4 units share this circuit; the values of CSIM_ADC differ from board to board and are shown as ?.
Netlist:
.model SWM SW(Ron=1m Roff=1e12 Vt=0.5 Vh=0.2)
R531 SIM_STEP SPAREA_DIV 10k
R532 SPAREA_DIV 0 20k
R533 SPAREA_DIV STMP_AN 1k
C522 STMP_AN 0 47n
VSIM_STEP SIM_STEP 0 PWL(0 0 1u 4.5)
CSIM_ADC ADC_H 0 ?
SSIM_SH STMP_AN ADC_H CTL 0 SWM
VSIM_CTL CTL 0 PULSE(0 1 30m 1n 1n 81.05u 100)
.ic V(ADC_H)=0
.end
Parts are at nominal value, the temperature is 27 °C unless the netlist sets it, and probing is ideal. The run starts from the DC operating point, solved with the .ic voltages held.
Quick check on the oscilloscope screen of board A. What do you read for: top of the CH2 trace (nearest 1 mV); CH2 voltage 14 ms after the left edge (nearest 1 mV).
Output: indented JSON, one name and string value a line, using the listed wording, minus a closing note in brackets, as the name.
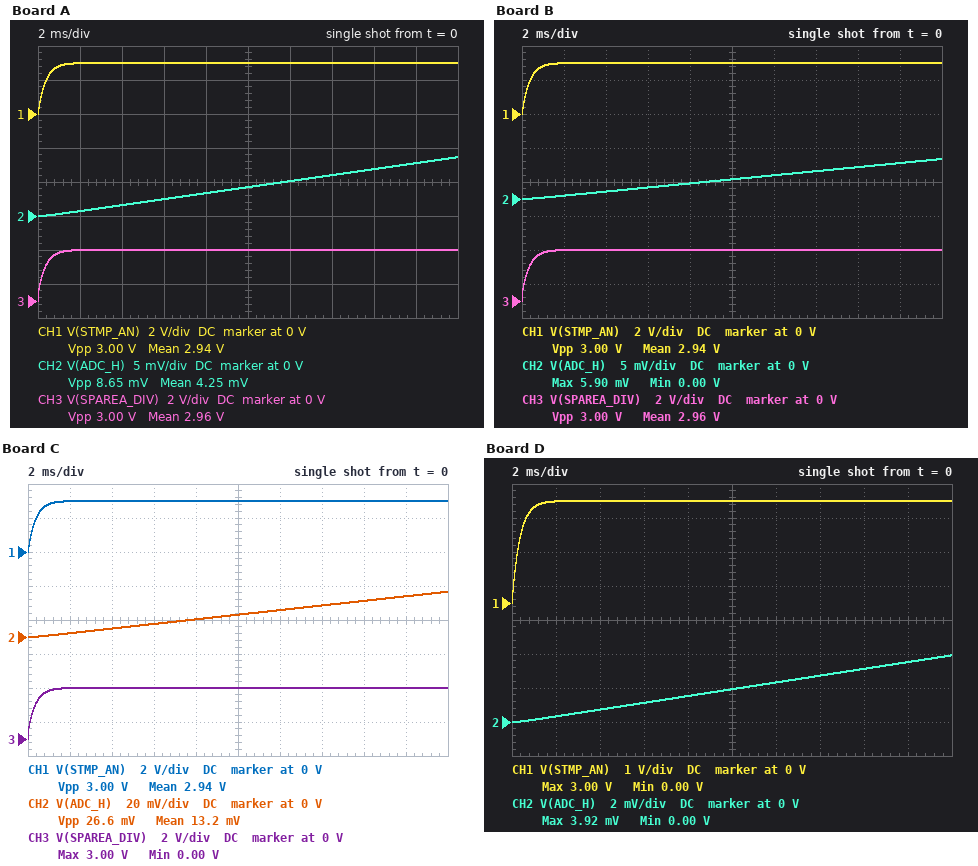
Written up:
{
  "top of the CH2 trace": "9 mV",
  "CH2 voltage 14 ms after the left edge": "6 mV"
}
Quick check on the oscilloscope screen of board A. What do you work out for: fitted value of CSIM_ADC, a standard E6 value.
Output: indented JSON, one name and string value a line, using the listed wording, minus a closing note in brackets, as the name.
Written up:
{
  "fitted value of CSIM_ADC, a standard E6 value": "6.8 pF"
}
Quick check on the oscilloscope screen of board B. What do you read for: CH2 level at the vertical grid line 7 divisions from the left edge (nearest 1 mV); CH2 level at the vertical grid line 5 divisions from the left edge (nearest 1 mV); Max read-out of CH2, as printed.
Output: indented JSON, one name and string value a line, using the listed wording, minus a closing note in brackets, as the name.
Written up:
{
  "CH2 level at the vertical grid line 7 divisions from the left edge": "4 mV",
  "CH2 level at the vertical grid line 5 divisions from the left edge": "3 mV",
  "Max read-out of CH2, as printed": "5.90 mV"
}
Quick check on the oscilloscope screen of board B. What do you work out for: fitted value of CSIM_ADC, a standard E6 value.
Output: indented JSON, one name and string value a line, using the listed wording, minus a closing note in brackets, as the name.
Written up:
{
  "fitted value of CSIM_ADC, a standard E6 value": "10 pF"
}
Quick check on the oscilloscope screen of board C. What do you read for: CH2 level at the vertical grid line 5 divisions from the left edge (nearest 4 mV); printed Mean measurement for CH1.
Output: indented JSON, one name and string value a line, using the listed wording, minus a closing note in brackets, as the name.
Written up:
{
  "CH2 level at the vertical grid line 5 divisions from the left edge": "12 mV",
  "printed Mean measurement for CH1": "2.94 V"
}
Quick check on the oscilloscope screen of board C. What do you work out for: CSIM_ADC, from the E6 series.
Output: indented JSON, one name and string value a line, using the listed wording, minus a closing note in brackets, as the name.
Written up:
{
  "CSIM_ADC, from the E6 series": "2.2 pF"
}
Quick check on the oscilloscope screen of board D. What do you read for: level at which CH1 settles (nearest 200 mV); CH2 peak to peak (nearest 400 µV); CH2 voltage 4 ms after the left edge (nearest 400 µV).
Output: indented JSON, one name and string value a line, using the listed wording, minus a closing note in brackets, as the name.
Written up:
{
  "level at which CH1 settles": "3.0 V",
  "CH2 peak to peak": "4.0 mV",
  "CH2 voltage 4 ms after the left edge": "800 µV"
}
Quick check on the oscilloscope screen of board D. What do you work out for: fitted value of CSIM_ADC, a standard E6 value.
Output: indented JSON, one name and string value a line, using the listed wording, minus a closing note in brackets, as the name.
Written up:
{
  "fitted value of CSIM_ADC, a standard E6 value": "15 pF"
}
